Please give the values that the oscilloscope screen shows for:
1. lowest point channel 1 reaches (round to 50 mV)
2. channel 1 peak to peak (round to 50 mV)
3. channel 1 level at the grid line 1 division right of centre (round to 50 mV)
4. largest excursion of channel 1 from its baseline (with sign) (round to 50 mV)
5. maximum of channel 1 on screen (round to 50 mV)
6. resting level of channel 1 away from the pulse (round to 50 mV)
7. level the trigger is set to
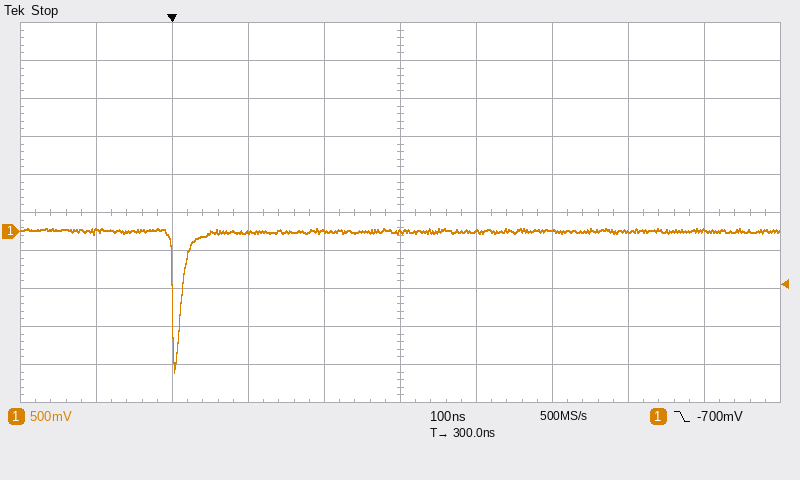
-1.85 V
1.90 V
0 mV
-1.85 V
50 mV
0 mV
-700 mV
